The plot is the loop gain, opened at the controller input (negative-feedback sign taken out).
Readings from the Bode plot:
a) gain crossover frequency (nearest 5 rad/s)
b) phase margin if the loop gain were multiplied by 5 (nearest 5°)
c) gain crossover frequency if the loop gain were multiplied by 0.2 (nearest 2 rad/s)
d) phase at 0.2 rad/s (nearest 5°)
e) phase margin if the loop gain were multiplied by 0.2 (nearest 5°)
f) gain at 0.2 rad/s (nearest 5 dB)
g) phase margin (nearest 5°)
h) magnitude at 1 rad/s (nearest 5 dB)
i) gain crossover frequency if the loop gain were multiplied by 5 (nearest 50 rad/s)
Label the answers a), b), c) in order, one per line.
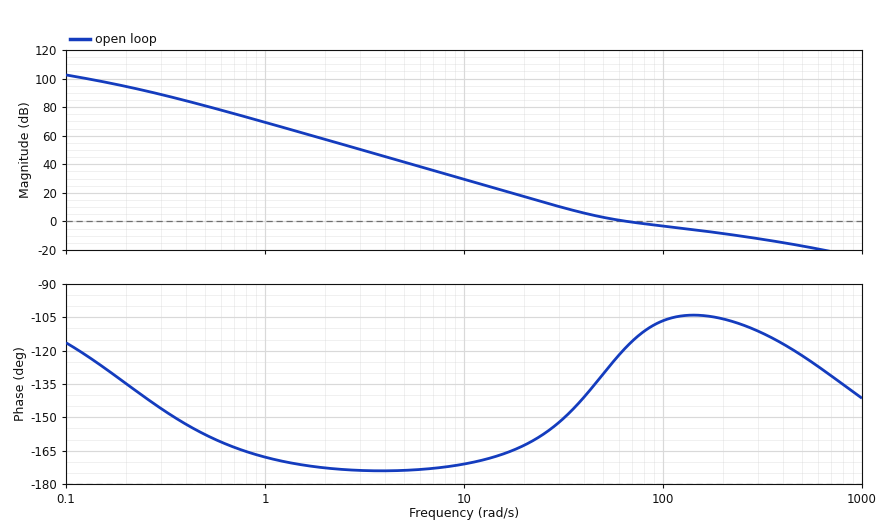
a) 65 rad/s
b) 65°
c) 24 rad/s
d) -135°
e) 20°
f) 95 dB
g) 60°
h) 70 dB
i) 350 rad/s
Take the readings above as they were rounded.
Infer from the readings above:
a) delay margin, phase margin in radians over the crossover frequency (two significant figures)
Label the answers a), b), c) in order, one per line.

a) 0.016 s
